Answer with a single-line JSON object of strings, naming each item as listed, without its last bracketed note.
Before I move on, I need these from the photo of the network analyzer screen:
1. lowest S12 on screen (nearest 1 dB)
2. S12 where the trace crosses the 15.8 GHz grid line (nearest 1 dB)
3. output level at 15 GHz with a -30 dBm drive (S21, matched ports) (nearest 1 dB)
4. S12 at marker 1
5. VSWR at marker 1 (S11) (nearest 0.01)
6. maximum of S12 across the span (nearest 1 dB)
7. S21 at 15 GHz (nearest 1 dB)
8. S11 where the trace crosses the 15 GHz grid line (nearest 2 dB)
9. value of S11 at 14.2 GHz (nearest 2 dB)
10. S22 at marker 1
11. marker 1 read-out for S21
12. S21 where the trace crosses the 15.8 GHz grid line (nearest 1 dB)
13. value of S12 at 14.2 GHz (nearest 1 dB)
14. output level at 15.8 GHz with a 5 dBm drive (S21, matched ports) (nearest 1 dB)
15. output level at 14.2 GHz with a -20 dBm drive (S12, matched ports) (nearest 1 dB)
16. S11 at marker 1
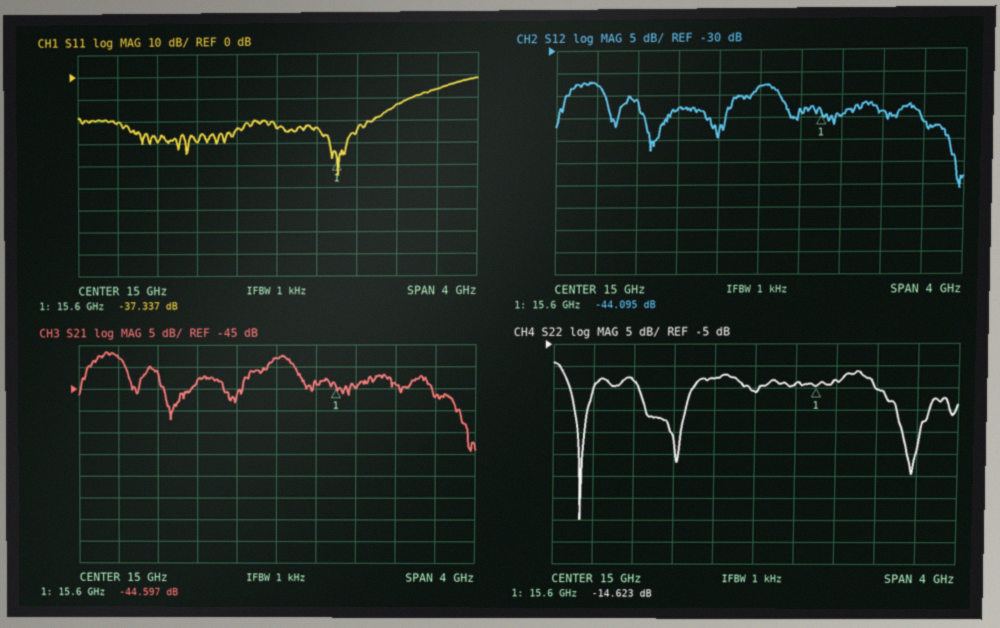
{"lowest S12 on screen": "-61 dB", "S12 where the trace crosses the 15.8 GHz grid line": "-45 dB", "output level at 15 GHz with a -30 dBm drive (S21, matched ports)": "-68 dBm", "S12 at marker 1": "-44.095 dB", "VSWR at marker 1 (S11)": "1.03", "maximum of S12 across the span": "-37 dB", "S21 at 15 GHz": "-38 dB", "S11 where the trace crosses the 15 GHz grid line": "-24 dB", "value of S11 at 14.2 GHz": "-30 dB", "S22 at marker 1": "-14.623 dB", "marker 1 read-out for S21": "-44.597 dB", "S21 where the trace crosses the 15.8 GHz grid line": "-45 dB", "value of S12 at 14.2 GHz": "-43 dB", "output level at 15.8 GHz with a 5 dBm drive (S21, matched ports)": "-40 dBm", "output level at 14.2 GHz with a -20 dBm drive (S12, matched ports)": "-63 dBm", "S11 at marker 1": "-37.337 dB"}
